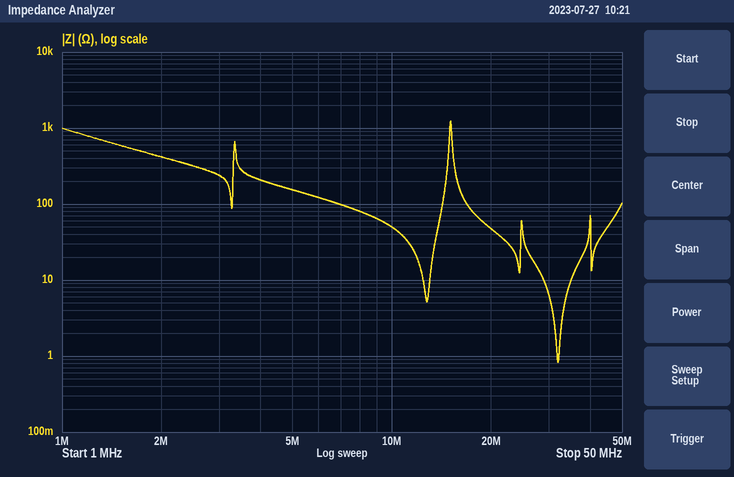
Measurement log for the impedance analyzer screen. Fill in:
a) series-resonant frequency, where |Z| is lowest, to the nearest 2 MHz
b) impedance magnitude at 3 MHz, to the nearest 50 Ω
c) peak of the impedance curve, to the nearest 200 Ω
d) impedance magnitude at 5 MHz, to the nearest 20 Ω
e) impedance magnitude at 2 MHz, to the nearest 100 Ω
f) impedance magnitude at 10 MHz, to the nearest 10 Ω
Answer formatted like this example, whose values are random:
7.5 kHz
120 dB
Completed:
32 MHz
250 Ω
1.2 kΩ
160 Ω
400 Ω
50 Ω
